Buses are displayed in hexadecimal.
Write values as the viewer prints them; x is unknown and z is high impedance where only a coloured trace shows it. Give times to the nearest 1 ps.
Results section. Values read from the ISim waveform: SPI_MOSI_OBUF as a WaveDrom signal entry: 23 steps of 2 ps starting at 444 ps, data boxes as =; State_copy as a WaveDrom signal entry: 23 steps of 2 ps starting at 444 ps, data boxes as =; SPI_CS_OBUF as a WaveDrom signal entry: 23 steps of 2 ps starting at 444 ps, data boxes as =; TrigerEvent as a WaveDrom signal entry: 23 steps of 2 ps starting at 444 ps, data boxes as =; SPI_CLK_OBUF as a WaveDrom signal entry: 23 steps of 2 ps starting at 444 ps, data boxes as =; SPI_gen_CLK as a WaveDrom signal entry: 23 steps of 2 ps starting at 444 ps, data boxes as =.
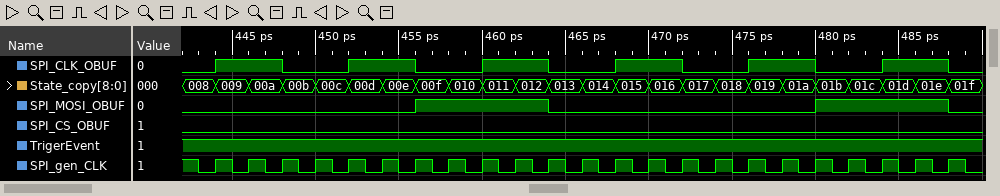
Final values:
{name: 'SPI_MOSI_OBUF', wave: '0.....1...0.......1...0'}
{name: 'State_copy', wave: '=======================', data: '009 00a 00b 00c 00d 00e 00f 010 011 012 013 014 015 016 017 018 019 01a 01b 01c 01d 01e 01f'}
{name: 'SPI_CS_OBUF', wave: '0......................'}
{name: 'TrigerEvent', wave: '1......................'}
{name: 'SPI_CLK_OBUF', wave: '1.0.1.0.1.0.1.0.1.0.1.0'}
{name: 'SPI_gen_CLK', wave: 'p......................'}
